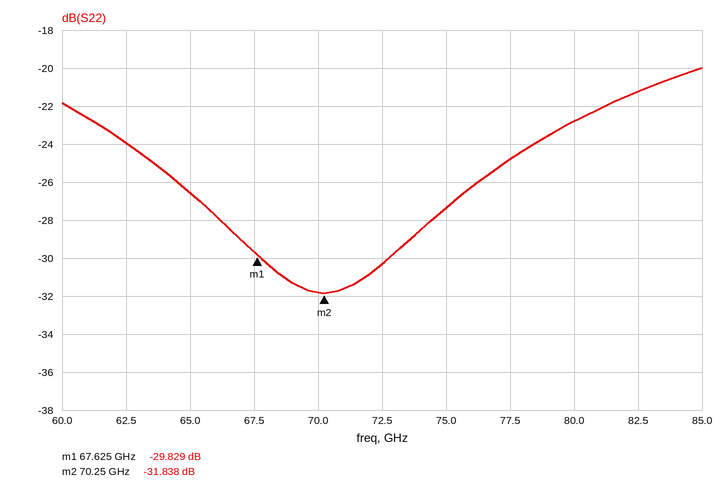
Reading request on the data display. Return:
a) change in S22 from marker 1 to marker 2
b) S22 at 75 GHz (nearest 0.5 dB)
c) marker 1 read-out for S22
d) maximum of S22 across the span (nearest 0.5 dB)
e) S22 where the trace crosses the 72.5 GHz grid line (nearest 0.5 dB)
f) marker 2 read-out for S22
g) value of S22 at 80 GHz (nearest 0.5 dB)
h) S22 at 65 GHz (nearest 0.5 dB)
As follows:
-2.009 dB
-27.5 dB
-29.829 dB
-20.0 dB
-30.5 dB
-31.838 dB
-23.0 dB
-26.5 dB
